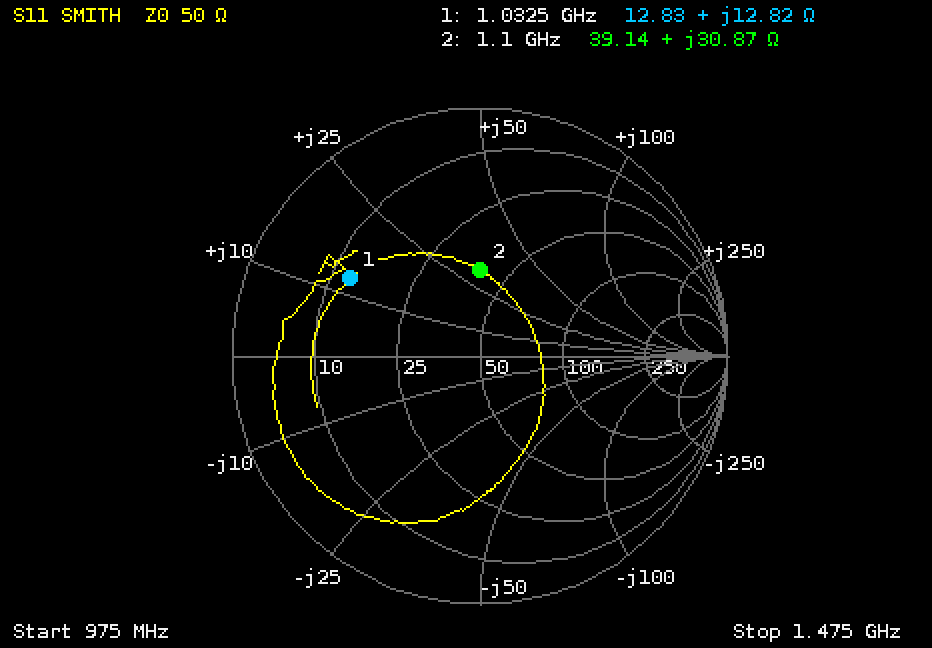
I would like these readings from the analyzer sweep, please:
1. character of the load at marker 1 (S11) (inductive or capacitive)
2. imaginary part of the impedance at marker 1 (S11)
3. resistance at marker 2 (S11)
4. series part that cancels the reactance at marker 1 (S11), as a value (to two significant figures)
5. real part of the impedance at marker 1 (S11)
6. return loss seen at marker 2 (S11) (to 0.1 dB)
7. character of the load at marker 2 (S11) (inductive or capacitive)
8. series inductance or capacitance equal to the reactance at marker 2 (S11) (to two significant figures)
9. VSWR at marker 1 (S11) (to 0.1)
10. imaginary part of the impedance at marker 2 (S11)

inductive
+12.82 Ω
39.14 Ω
12 pF
12.83 Ω
9.2 dB
inductive
4.5 nH
4.2
+30.87 Ω
